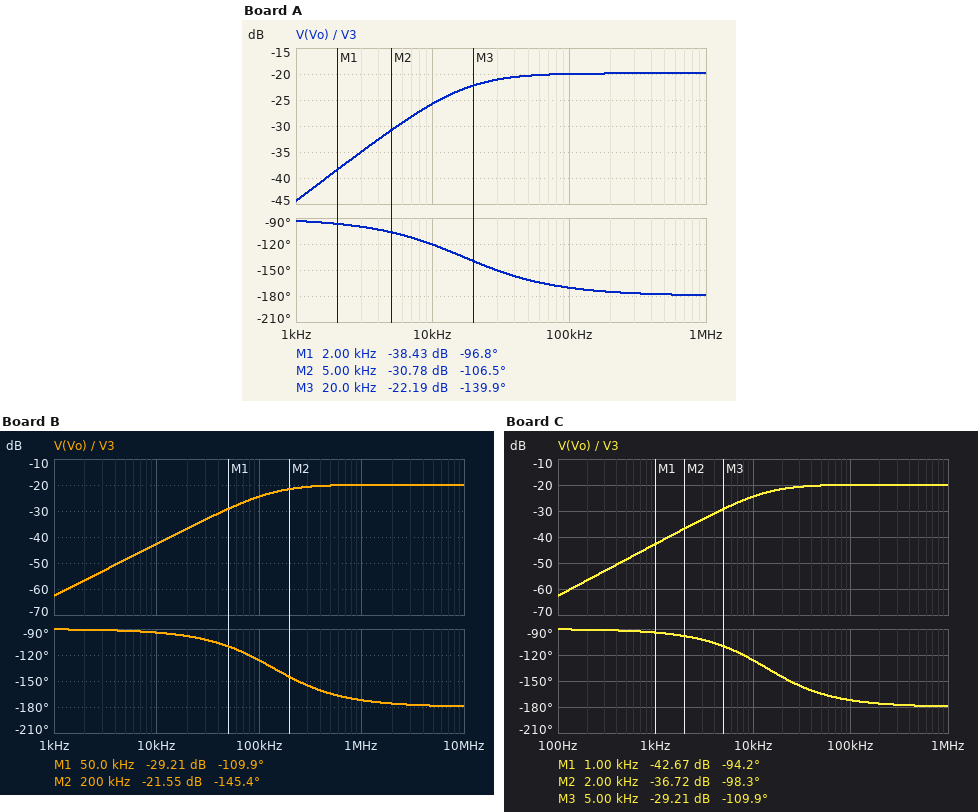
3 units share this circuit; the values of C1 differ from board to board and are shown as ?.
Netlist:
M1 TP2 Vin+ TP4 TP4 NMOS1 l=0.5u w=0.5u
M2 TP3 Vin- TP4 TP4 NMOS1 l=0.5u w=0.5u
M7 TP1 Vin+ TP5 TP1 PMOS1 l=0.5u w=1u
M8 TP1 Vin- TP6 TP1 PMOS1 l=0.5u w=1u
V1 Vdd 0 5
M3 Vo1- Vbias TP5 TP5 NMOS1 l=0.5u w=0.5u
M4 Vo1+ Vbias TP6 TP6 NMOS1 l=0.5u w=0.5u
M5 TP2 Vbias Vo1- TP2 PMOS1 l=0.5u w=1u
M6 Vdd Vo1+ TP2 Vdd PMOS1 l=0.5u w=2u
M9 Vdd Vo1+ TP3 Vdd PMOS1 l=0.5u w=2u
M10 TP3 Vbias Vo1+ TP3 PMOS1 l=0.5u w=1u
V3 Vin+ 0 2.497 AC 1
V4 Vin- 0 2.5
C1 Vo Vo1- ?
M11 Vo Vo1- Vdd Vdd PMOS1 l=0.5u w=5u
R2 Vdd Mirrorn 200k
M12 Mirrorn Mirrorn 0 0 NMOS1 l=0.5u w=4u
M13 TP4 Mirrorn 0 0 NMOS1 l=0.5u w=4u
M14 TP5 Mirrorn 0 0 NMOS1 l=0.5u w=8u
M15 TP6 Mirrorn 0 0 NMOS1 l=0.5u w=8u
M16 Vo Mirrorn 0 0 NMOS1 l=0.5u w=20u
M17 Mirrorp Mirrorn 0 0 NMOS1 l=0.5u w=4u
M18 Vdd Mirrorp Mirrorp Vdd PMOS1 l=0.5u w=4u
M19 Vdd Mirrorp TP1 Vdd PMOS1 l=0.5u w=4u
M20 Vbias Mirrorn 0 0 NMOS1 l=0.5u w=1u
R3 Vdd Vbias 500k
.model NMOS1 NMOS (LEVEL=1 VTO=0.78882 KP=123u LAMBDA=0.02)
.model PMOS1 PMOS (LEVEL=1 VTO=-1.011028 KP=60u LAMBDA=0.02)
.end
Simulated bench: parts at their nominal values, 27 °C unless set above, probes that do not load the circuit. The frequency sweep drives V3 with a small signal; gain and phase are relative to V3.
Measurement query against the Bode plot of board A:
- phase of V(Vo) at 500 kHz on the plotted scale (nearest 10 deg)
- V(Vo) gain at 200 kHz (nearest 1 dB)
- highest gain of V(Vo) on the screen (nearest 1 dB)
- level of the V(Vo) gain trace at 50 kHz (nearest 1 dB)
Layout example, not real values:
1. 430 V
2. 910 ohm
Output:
1. -180 deg
2. -20 dB
3. -20 dB
4. -20 dB
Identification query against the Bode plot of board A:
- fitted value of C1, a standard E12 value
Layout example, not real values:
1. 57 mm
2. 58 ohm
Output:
1. 18 pF
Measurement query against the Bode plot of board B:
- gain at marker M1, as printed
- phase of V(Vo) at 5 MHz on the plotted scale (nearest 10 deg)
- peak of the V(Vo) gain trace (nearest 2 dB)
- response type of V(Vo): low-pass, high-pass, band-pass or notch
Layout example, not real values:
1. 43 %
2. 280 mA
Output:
1. -29.21 dB
2. -180 deg
3. -20 dB
4. high-pass
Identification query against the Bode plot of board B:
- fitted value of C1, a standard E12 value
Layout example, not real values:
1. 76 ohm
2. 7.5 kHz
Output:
1. 2.2 pF
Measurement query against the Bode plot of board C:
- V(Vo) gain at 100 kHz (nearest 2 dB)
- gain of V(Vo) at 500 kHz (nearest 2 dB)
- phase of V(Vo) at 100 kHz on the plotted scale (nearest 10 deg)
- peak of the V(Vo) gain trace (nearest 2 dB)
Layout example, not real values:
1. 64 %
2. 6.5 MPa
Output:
1. -20 dB
2. -20 dB
3. -170 deg
4. -20 dB
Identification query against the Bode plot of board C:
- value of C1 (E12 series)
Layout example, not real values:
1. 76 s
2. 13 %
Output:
1. 22 pF
